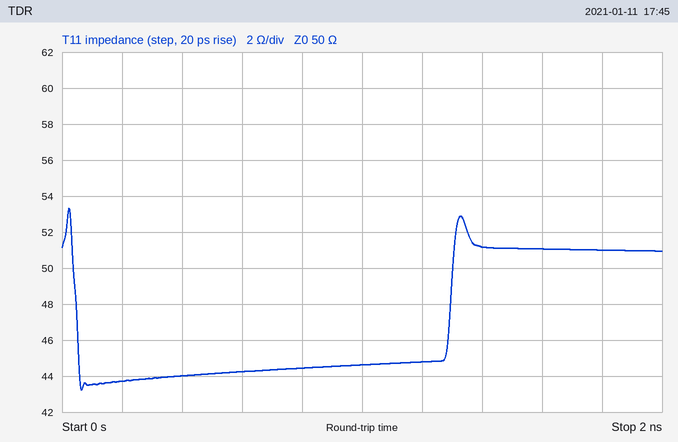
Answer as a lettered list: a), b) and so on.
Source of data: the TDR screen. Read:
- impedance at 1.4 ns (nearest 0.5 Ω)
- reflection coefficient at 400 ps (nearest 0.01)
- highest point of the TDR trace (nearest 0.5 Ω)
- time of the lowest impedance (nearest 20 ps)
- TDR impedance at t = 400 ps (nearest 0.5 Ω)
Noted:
a) 51.0 Ω
b) -0.06
c) 53.5 Ω
d) 60 ps
e) 44.0 Ω
